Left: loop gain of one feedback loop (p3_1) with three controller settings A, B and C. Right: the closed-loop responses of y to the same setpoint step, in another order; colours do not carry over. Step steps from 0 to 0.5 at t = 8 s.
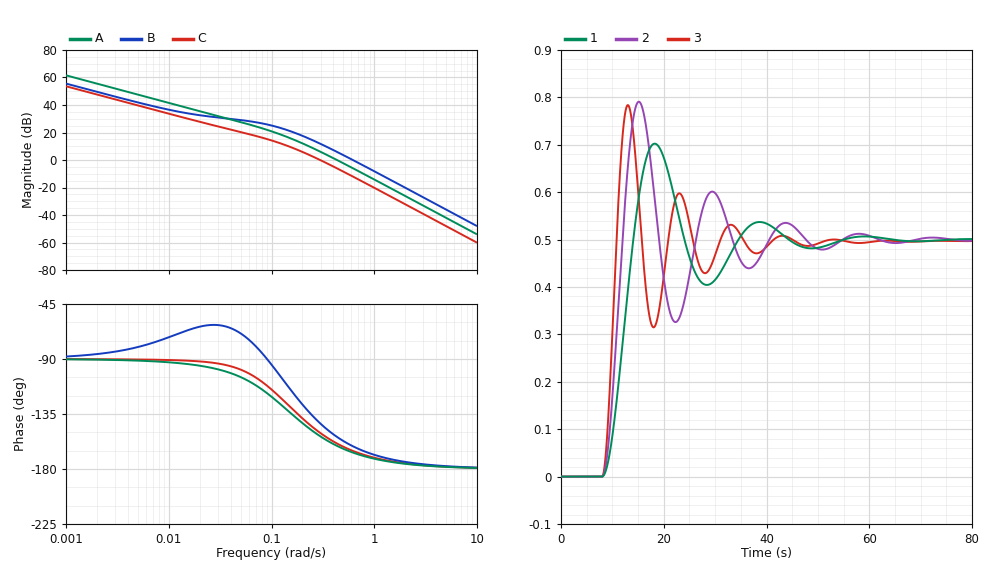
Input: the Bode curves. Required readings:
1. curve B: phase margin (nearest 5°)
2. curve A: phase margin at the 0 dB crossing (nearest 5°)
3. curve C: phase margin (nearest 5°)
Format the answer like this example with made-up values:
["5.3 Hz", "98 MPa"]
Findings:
["20°", "20°", "30°"]
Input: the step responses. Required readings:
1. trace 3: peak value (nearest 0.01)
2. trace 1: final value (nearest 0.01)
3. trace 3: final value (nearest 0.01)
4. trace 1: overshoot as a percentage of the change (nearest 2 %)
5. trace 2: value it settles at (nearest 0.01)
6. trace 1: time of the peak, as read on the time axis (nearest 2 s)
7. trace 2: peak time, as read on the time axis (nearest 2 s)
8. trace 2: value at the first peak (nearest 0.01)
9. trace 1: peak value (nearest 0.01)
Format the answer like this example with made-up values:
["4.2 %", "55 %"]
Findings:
["0.78", "0.50", "0.50", "40 %", "0.50", "18 s", "16 s", "0.79", "0.70"]
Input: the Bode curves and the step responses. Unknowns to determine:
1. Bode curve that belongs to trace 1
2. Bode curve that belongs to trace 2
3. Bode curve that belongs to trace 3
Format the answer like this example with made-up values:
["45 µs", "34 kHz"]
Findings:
["C", "A", "B"]
